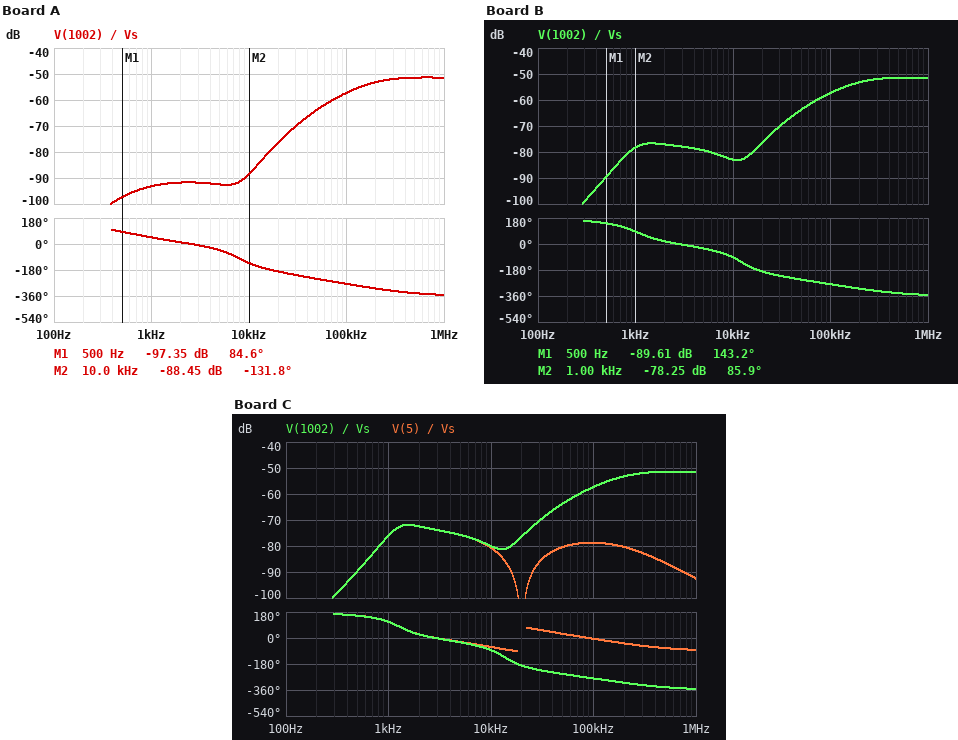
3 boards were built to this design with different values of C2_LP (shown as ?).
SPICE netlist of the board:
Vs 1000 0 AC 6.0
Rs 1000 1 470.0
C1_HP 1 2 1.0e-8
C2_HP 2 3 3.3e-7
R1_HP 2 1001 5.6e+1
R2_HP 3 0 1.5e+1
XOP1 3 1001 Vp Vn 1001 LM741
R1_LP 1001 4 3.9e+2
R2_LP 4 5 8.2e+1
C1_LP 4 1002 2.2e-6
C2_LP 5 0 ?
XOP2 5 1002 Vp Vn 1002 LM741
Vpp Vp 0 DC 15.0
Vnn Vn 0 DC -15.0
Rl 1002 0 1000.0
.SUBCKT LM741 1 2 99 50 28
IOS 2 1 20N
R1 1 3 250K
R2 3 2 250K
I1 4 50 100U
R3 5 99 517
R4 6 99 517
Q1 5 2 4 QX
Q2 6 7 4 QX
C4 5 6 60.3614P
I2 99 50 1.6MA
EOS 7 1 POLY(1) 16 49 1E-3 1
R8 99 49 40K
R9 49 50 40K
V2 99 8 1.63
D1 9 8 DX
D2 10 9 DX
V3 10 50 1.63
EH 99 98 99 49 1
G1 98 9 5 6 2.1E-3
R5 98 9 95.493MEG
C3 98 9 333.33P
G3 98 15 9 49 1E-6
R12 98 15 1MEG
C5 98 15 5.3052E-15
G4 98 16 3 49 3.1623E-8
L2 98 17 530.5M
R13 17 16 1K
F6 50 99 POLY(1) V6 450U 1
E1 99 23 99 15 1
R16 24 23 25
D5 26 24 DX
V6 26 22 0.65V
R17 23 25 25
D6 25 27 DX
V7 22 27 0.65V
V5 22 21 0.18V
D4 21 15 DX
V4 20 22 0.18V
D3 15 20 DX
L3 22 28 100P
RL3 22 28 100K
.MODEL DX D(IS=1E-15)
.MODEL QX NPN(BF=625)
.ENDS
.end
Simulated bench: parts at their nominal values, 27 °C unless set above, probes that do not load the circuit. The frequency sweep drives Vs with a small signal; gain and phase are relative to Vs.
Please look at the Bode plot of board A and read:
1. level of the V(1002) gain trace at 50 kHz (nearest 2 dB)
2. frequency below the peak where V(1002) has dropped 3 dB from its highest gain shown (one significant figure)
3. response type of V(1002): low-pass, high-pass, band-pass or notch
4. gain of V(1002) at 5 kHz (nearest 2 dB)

-64 dB
200 kHz
high-pass
-92 dB
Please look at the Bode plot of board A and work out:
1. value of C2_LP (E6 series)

1.5 µF
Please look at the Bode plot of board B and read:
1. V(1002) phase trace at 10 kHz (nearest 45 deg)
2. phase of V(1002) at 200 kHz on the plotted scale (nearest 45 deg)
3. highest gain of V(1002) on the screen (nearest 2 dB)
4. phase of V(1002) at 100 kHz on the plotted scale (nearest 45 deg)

-90 deg
-315 deg
-52 dB
-270 deg
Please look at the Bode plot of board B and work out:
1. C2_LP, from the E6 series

330 nF
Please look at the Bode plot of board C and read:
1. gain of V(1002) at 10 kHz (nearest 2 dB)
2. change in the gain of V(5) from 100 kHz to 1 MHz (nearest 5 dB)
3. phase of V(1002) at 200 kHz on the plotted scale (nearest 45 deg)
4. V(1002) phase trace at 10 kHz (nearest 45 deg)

-80 dB
-15 dB
-315 deg
-90 deg
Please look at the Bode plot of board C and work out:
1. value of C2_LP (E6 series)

220 nF
